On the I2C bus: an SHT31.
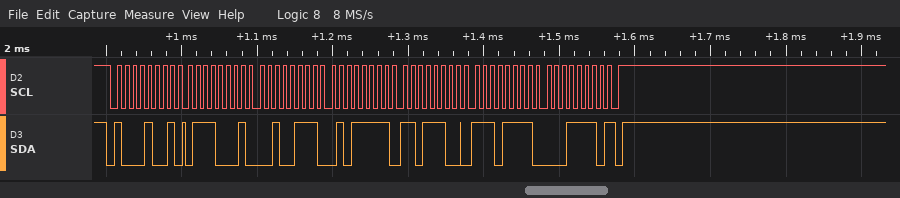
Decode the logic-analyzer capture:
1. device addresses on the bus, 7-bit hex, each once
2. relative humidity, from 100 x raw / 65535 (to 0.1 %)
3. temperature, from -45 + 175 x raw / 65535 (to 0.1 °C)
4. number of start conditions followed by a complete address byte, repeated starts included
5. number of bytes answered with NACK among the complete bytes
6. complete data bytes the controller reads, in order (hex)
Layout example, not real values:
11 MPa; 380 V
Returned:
0x44; 86.3 %; 32.4 °C; 1; 1; 71 27 5F DC EF 1E
